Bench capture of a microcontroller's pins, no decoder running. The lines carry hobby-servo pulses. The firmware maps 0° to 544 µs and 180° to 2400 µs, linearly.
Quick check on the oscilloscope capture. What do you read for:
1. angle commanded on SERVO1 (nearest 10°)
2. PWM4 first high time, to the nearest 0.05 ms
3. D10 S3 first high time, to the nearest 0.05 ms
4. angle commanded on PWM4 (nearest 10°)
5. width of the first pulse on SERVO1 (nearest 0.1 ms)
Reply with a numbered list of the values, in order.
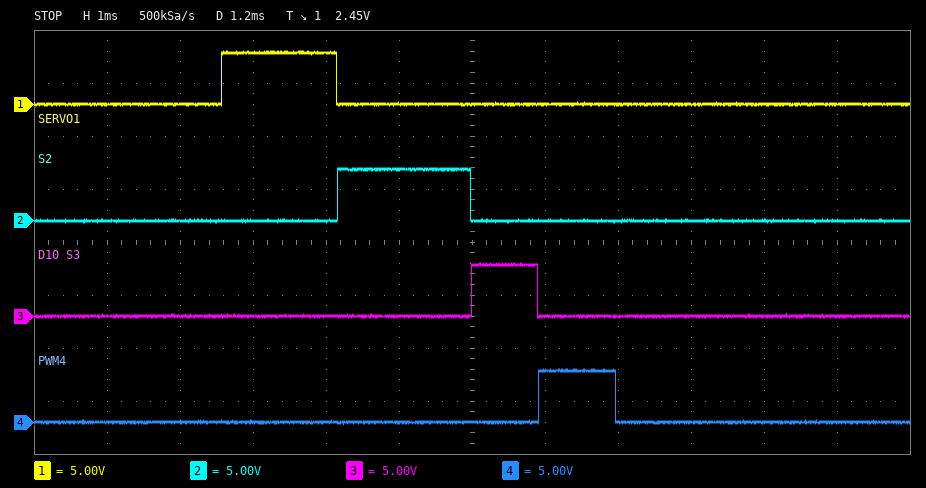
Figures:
1. 100°
2. 1.05 ms
3. 0.90 ms
4. 50°
5. 1.6 ms
